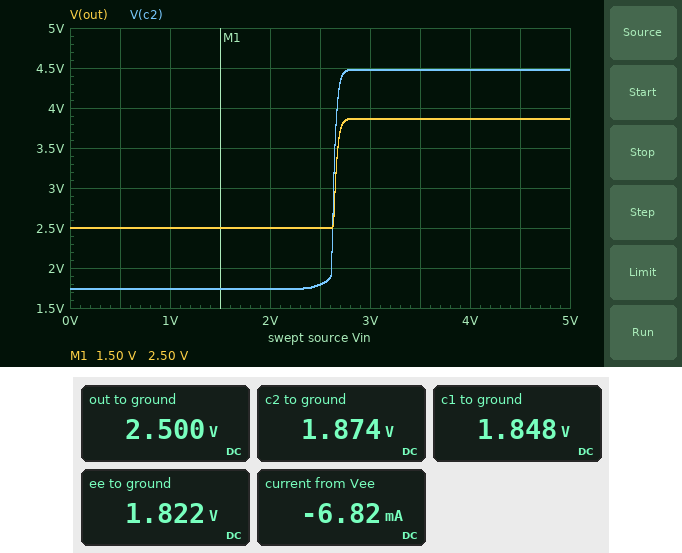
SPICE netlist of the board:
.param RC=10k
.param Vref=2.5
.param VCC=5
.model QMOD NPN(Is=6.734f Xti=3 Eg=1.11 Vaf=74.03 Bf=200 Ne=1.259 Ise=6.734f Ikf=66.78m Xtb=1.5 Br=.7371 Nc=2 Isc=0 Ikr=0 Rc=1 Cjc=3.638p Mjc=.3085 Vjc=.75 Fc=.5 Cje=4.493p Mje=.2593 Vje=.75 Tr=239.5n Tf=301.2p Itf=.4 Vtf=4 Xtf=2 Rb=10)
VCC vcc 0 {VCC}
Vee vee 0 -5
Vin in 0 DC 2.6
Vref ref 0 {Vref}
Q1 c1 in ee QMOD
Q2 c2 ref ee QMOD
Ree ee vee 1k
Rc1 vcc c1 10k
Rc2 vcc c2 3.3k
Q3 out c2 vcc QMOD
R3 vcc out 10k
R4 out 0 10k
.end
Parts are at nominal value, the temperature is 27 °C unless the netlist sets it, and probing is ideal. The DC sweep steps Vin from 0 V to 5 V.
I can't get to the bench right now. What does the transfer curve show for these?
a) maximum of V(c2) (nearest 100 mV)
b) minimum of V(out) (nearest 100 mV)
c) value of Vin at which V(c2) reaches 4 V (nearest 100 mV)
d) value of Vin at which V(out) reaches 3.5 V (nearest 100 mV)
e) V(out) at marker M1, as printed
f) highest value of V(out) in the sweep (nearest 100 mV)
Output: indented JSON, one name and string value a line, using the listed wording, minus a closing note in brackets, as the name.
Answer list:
{
  "maximum of V(c2)": "4.5 V",
  "minimum of V(out)": "2.5 V",
  "value of Vin at which V(c2) reaches 4 V": "2.7 V",
  "value of Vin at which V(out) reaches 3.5 V": "2.7 V",
  "V(out) at marker M1, as printed": "2.50 V",
  "highest value of V(out) in the sweep": "3.9 V"
}
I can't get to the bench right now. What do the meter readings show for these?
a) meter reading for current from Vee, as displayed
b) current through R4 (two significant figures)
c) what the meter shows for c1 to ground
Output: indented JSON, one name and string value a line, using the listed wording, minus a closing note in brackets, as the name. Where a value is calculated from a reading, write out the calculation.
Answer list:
{
  "meter reading for current from Vee, as displayed": "-6.82 mA",
  "current through R4": "(2.5 V) / 10 kΩ = 250 µA",
  "what the meter shows for c1 to ground": "1.848 V"
}
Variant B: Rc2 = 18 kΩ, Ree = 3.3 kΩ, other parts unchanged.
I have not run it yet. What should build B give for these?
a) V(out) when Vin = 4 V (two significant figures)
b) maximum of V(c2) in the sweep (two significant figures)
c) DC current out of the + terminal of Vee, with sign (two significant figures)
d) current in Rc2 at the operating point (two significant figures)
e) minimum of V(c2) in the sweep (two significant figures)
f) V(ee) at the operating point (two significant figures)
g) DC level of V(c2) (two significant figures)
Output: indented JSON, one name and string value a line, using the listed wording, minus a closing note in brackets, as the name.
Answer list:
{
  "V(out) when Vin = 4 V": "3.1 V",
  "maximum of V(c2) in the sweep": "3.7 V",
  "DC current out of the + terminal of Vee, with sign": "-2.1 mA",
  "current in Rc2 at the operating point": "130 µA",
  "minimum of V(c2) in the sweep": "1.8 V",
  "V(ee) at the operating point": "1.9 V",
  "DC level of V(c2)": "2.7 V"
}
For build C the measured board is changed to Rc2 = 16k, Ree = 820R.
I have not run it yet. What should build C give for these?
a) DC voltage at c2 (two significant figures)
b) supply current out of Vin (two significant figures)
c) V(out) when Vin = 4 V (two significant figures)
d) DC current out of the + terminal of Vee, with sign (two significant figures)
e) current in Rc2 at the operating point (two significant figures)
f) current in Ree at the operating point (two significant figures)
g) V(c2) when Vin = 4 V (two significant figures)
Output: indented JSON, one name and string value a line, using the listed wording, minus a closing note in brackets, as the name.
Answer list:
{
  "DC voltage at c2": "1.8 V",
  "supply current out of Vin": "6.6 mA",
  "V(out) when Vin = 4 V": "3.2 V",
  "DC current out of the + terminal of Vee, with sign": "-8.3 mA",
  "current in Rc2 at the operating point": "200 µA",
  "current in Ree at the operating point": "8.3 mA",
  "V(c2) when Vin = 4 V": "3.8 V"
}
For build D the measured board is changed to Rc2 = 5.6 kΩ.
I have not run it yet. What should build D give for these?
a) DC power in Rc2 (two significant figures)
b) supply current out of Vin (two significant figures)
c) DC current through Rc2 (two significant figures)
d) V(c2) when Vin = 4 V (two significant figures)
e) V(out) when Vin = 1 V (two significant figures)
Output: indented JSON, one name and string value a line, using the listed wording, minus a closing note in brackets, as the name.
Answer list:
{
  "DC power in Rc2": "1.8 mW",
  "supply current out of Vin": "5.4 mA",
  "DC current through Rc2": "560 µA",
  "V(c2) when Vin = 4 V": "4.3 V",
  "V(out) when Vin = 1 V": "2.5 V"
}
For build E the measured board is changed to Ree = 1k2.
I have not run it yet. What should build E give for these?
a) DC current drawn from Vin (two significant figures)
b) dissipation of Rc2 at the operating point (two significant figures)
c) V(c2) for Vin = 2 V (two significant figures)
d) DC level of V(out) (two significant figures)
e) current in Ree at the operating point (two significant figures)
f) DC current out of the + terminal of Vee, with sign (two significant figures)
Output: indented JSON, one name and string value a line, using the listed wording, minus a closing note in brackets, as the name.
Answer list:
{
  "DC current drawn from Vin": "4.4 mA",
  "dissipation of Rc2 at the operating point": "2.8 mW",
  "V(c2) for Vin = 2 V": "1.8 V",
  "DC level of V(out)": "2.5 V",
  "current in Ree at the operating point": "5.7 mA",
  "DC current out of the + terminal of Vee, with sign": "-5.7 mA"
}
